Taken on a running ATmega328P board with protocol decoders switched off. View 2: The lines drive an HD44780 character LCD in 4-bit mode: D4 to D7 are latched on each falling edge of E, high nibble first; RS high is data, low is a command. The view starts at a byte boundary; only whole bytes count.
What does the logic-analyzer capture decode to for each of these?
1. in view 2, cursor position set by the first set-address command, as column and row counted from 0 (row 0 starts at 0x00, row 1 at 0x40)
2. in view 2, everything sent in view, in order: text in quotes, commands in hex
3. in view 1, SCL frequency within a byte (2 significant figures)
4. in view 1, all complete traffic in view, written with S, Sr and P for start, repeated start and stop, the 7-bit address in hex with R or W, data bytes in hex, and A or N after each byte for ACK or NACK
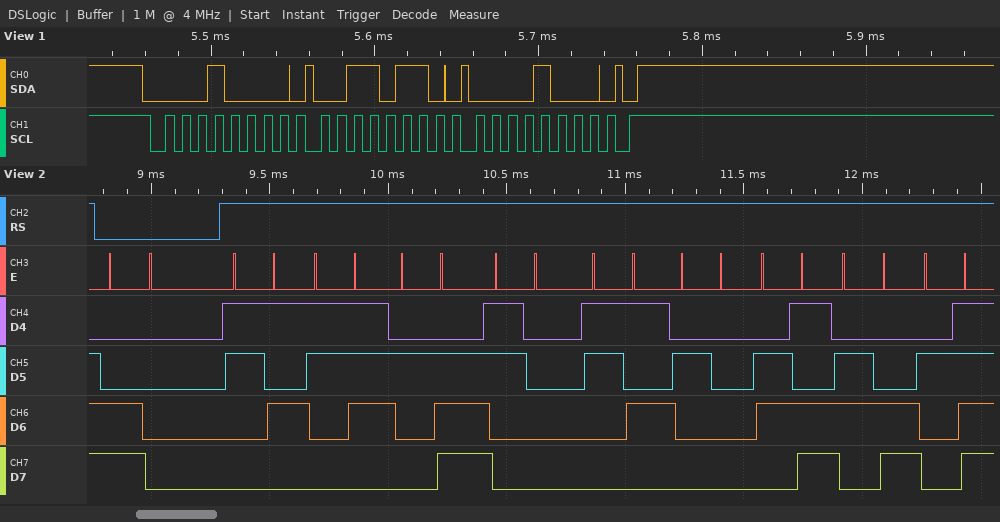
column 0, row 1
0xC0 "57.05 ml/"
100 kHz
S 08W A 36 A 08 A P
